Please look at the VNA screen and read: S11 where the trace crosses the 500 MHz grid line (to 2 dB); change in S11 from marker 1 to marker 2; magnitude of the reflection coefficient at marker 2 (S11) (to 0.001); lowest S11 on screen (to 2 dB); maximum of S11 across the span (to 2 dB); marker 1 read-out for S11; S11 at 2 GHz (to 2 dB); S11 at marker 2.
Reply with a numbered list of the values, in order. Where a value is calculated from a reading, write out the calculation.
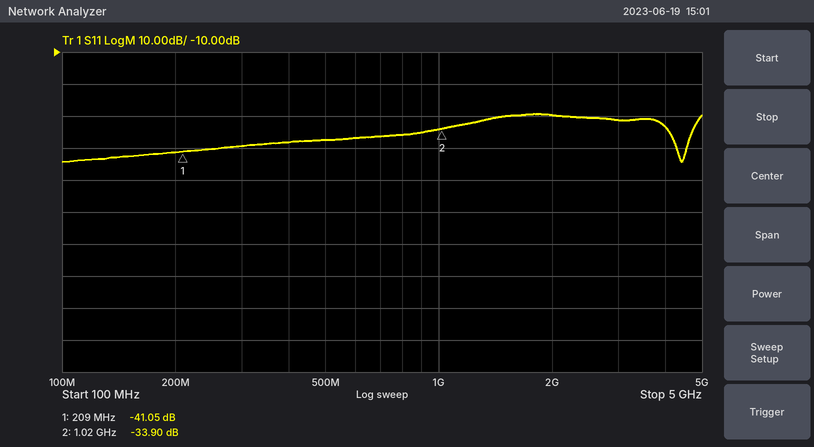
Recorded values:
1. -38 dB
2. -33.9 − (-41.05) = 7.15 dB
3. 10^(-33.9/20) ≈ 0.020
4. -44 dB
5. -30 dB
6. -41.05 dB
7. -30 dB
8. -33.90 dB
